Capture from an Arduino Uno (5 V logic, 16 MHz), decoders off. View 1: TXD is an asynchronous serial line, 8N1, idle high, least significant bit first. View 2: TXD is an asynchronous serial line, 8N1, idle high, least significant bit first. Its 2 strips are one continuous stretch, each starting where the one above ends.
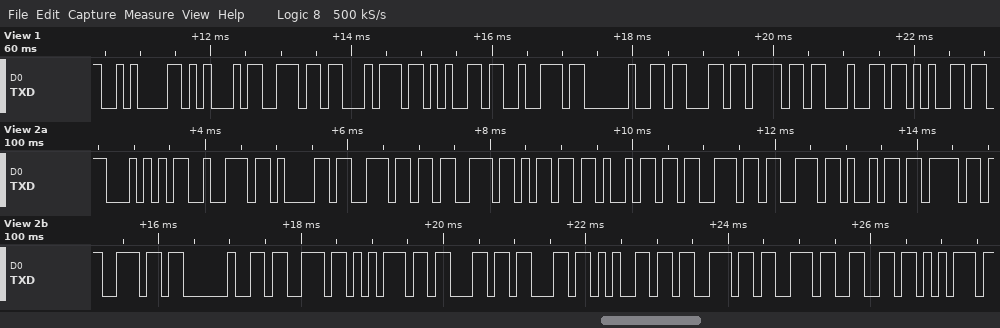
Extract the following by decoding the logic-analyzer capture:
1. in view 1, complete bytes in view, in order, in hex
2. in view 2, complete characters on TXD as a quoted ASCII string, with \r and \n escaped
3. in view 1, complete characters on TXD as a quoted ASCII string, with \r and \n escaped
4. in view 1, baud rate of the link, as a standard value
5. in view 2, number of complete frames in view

0x0A 0x45 0x6E 0x74 0x65 0x72 0x20 0x63 0x6F 0x64 0x65
"Transmission successfu"
"\nEnter code"
9600 baud
22
